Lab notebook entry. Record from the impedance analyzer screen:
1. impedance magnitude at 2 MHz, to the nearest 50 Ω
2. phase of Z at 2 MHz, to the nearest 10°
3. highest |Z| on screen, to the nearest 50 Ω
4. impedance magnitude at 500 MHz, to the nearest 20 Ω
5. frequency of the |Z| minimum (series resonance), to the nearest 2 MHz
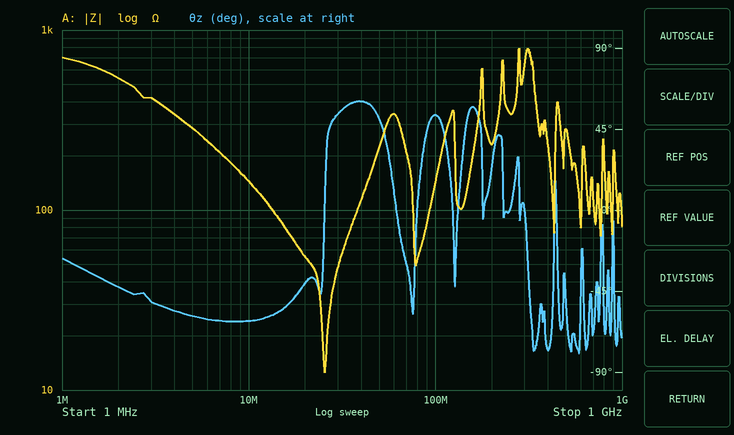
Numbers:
550 Ω
-40°
800 Ω
280 Ω
26 MHz
